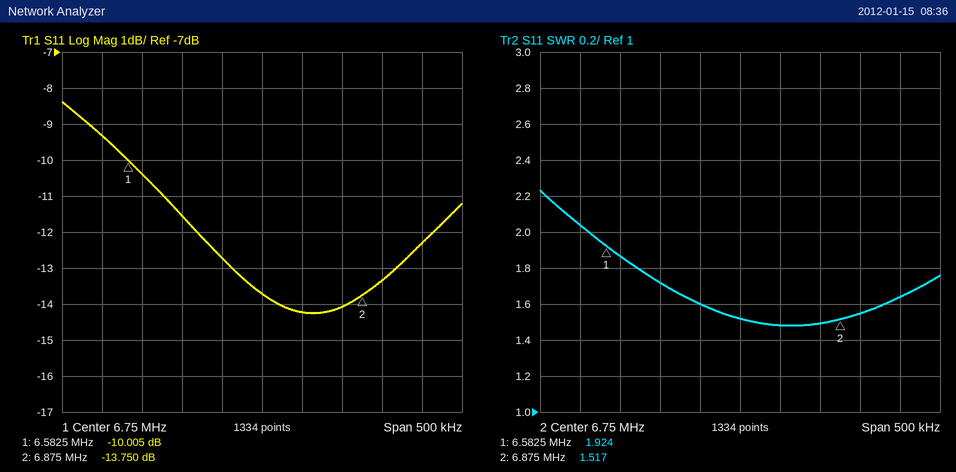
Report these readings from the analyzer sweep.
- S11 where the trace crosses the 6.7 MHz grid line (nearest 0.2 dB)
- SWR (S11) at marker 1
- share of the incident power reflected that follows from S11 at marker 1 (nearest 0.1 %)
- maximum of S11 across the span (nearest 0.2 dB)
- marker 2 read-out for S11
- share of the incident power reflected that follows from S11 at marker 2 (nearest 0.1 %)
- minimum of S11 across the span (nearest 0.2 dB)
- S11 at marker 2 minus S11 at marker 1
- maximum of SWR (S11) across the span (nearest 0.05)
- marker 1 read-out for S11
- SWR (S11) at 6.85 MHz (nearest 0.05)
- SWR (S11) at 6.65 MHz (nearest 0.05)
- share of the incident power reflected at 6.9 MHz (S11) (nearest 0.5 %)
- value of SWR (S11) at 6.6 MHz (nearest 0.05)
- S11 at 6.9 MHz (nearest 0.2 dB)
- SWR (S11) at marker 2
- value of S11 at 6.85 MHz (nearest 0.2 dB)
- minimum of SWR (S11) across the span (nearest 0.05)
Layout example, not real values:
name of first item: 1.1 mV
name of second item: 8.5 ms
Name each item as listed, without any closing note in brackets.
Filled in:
S11 where the trace crosses the 6.7 MHz grid line: -12.8 dB
SWR (S11) at marker 1: 1.924
share of the incident power reflected that follows from S11 at marker 1: 10.0 %
maximum of S11 across the span: -8.4 dB
marker 2 read-out for S11: -13.750 dB
share of the incident power reflected that follows from S11 at marker 2: 4.2 %
minimum of S11 across the span: -14.2 dB
S11 at marker 2 minus S11 at marker 1: -3.745 dB
maximum of SWR (S11) across the span: 2.25
marker 1 read-out for S11: -10.005 dB
SWR (S11) at 6.85 MHz: 1.50
SWR (S11) at 6.65 MHz: 1.70
share of the incident power reflected at 6.9 MHz (S11): 4.5 %
value of SWR (S11) at 6.6 MHz: 1.85
S11 at 6.9 MHz: -13.4 dB
SWR (S11) at marker 2: 1.517
value of S11 at 6.85 MHz: -14.0 dB
minimum of SWR (S11) across the span: 1.50
